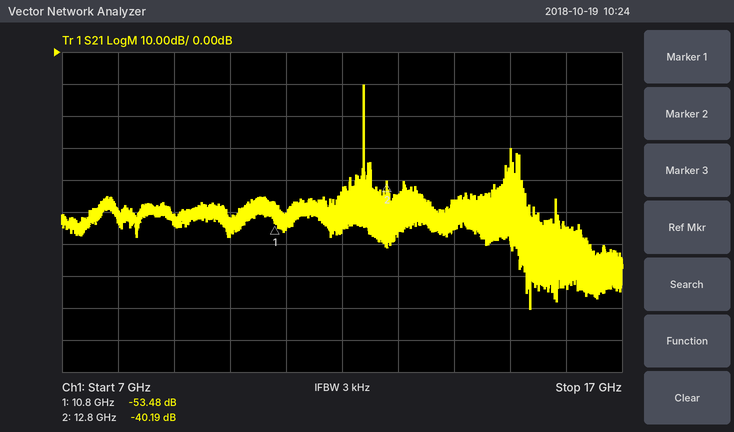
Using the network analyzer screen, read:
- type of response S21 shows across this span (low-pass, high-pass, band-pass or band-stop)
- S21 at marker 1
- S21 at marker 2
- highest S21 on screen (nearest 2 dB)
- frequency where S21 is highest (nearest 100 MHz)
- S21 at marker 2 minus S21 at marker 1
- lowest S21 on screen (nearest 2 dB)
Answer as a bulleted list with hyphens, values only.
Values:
- band-pass
- -53.48 dB
- -40.19 dB
- -10 dB
- 12.4 GHz
- 13.29 dB
- -80 dB
